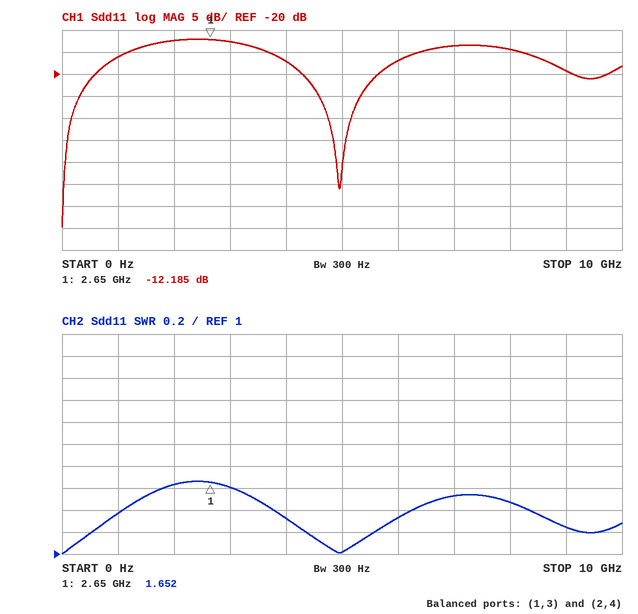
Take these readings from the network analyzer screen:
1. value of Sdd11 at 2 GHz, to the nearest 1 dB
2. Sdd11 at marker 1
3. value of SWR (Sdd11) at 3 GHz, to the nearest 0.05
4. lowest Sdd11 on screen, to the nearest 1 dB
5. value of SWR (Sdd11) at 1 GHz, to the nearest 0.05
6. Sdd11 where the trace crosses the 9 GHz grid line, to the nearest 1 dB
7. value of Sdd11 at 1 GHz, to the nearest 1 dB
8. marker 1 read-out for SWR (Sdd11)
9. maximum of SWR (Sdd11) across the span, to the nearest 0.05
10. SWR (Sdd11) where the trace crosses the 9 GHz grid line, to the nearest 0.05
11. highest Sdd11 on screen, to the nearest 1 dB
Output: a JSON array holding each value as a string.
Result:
["-12 dB", "-12.185 dB", "1.60", "-55 dB", "1.35", "-19 dB", "-16 dB", "1.652", "1.65", "1.25", "-12 dB"]
